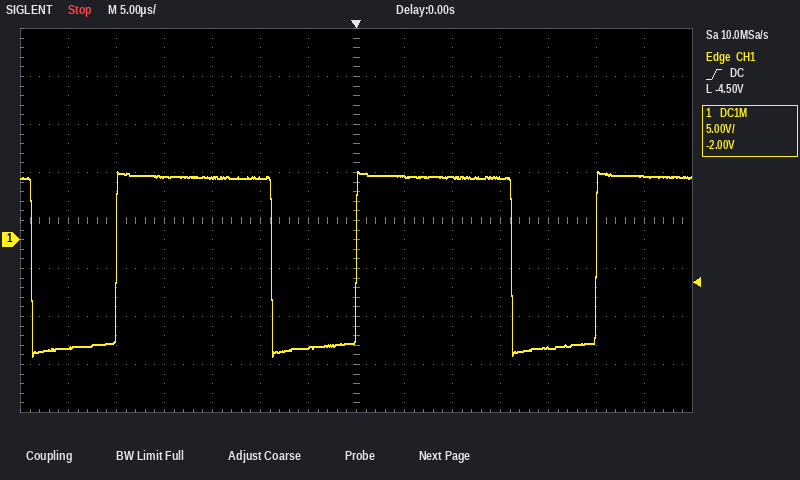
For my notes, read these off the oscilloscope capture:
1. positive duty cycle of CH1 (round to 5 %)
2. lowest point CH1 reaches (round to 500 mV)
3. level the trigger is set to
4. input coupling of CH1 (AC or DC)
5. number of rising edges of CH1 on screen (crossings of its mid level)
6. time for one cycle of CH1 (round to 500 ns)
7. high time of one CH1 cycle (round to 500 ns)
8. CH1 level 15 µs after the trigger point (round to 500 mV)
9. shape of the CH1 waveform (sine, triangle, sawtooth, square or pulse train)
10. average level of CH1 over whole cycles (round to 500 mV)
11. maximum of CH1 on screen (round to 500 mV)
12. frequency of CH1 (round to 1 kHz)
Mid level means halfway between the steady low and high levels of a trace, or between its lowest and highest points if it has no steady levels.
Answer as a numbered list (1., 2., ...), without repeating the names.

1. 65 %
2. -12.0 V
3. -4.50 V
4. DC
5. 3
6. 25.0 µs
7. 16.0 µs
8. 6.5 V
9. pulse train
10. 500 mV
11. 7.0 V
12. 40 kHz
